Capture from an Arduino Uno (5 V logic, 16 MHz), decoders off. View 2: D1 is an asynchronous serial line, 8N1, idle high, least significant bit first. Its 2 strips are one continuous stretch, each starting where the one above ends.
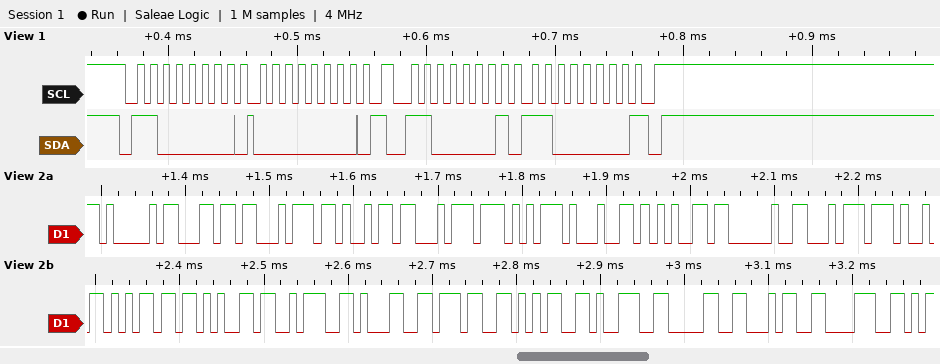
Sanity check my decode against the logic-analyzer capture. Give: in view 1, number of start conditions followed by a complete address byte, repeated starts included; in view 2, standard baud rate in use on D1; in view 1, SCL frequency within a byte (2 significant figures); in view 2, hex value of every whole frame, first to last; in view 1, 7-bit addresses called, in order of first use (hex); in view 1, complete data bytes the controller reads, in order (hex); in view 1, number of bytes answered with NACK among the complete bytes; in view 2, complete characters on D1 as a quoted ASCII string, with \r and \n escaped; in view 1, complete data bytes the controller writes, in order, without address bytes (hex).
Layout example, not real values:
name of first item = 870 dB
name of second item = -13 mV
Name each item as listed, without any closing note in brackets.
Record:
in view 1, number of start conditions followed by a complete address byte, repeated starts included = 2
in view 2, standard baud rate in use on D1 = 115200 baud
in view 1, SCL frequency within a byte = 100 kHz
in view 2, hex value of every whole frame, first to last = 41 6C 74 69 74 75 64 65 20 74 69 6D 65 3A 31 37 35 39 30 34 38
in view 1, 7-bit addresses called, in order of first use = 0x60
in view 1, complete data bytes the controller reads, in order = C0
in view 1, number of bytes answered with NACK among the complete bytes = 1
in view 2, complete characters on D1 as a quoted ASCII string, with \r and \n escaped = "Altitude time:1759048"
in view 1, complete data bytes the controller writes, in order, without address bytes = 00
